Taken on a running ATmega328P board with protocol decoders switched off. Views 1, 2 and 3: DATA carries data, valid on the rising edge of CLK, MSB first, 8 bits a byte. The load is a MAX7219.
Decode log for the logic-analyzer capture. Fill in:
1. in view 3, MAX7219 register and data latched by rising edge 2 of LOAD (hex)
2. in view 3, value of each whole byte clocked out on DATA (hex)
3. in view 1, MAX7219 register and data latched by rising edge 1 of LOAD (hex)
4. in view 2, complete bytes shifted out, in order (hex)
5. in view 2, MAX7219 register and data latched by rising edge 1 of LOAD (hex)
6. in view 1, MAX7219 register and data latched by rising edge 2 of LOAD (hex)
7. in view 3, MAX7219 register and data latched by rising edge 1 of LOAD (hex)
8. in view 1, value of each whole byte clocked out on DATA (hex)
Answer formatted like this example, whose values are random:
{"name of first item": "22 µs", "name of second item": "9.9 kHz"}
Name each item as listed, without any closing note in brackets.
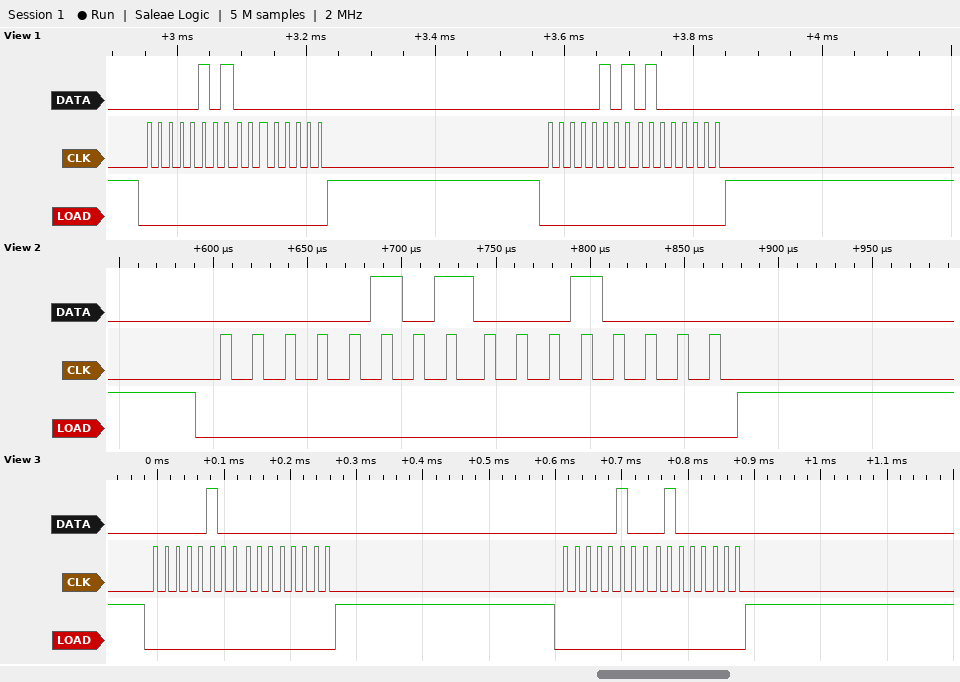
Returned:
{"in view 3, MAX7219 register and data latched by rising edge 2 of LOAD": "register 0x4, data 0x40", "in view 3, value of each whole byte clocked out on DATA": "04 00 04 40", "in view 1, MAX7219 register and data latched by rising edge 1 of LOAD": "register 0x5, data 0x00", "in view 2, complete bytes shifted out, in order": "05 10", "in view 2, MAX7219 register and data latched by rising edge 1 of LOAD": "register 0x5, data 0x10", "in view 1, MAX7219 register and data latched by rising edge 2 of LOAD": "register 0x5, data 0x40", "in view 3, MAX7219 register and data latched by rising edge 1 of LOAD": "register 0x4, data 0x00", "in view 1, value of each whole byte clocked out on DATA": "0x05 0x00 0x05 0x40"}
